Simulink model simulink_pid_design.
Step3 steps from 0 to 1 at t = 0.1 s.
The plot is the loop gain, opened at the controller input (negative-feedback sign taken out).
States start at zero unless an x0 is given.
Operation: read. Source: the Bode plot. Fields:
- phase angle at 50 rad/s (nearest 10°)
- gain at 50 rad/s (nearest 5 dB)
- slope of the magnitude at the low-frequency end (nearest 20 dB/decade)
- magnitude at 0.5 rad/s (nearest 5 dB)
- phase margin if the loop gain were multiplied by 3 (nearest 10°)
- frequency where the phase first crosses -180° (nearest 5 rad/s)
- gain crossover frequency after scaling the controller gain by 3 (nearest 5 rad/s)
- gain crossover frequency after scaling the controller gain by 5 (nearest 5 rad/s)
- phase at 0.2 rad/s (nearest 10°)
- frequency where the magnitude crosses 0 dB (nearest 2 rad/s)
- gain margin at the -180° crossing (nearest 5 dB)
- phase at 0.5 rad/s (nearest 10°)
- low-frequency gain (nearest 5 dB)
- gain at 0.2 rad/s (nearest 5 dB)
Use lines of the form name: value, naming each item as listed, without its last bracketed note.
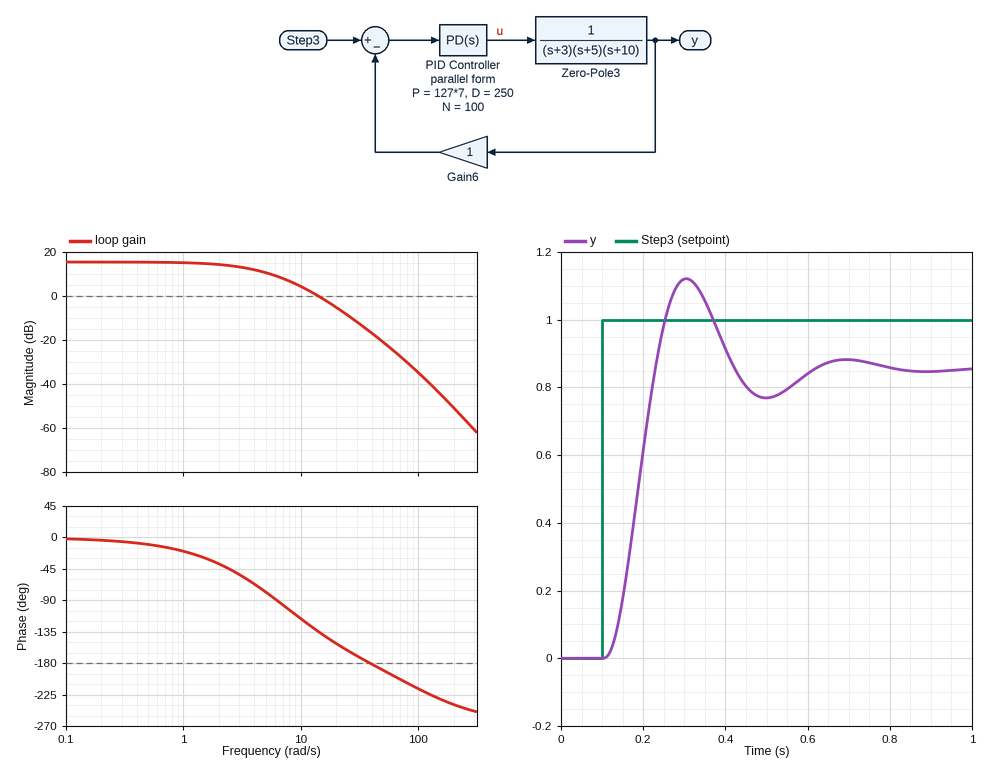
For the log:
phase angle at 50 rad/s: -190°
gain at 50 rad/s: -20 dB
slope of the magnitude at the low-frequency end: 0 dB/decade
magnitude at 0.5 rad/s: 15 dB
phase margin if the loop gain were multiplied by 3: 20°
frequency where the phase first crosses -180°: 40 rad/s
gain crossover frequency after scaling the controller gain by 3: 25 rad/s
gain crossover frequency after scaling the controller gain by 5: 35 rad/s
phase at 0.2 rad/s: 0°
frequency where the magnitude crosses 0 dB: 14 rad/s
gain margin at the -180° crossing: 15 dB
phase at 0.5 rad/s: -10°
low-frequency gain: 15 dB
gain at 0.2 rad/s: 15 dB
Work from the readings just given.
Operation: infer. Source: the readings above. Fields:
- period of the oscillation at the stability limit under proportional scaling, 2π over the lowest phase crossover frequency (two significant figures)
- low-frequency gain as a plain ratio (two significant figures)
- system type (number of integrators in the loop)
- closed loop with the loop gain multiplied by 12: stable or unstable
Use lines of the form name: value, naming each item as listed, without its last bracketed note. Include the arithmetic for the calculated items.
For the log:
period of the oscillation at the stability limit under proportional scaling, 2π over the lowest phase crossover frequency: 2π / 40 = 0.16 s
low-frequency gain as a plain ratio: 10^(15 / 20) = 5.6
system type: 0
closed loop with the loop gain multiplied by 12: stable or unstable: unstable
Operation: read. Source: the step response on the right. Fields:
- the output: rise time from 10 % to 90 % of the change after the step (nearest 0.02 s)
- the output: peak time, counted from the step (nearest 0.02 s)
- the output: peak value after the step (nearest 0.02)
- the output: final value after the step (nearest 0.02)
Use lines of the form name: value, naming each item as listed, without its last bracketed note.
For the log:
the output: rise time from 10 % to 90 % of the change after the step: 0.08 s
the output: peak time, counted from the step: 0.20 s
the output: peak value after the step: 1.12
the output: final value after the step: 0.86
